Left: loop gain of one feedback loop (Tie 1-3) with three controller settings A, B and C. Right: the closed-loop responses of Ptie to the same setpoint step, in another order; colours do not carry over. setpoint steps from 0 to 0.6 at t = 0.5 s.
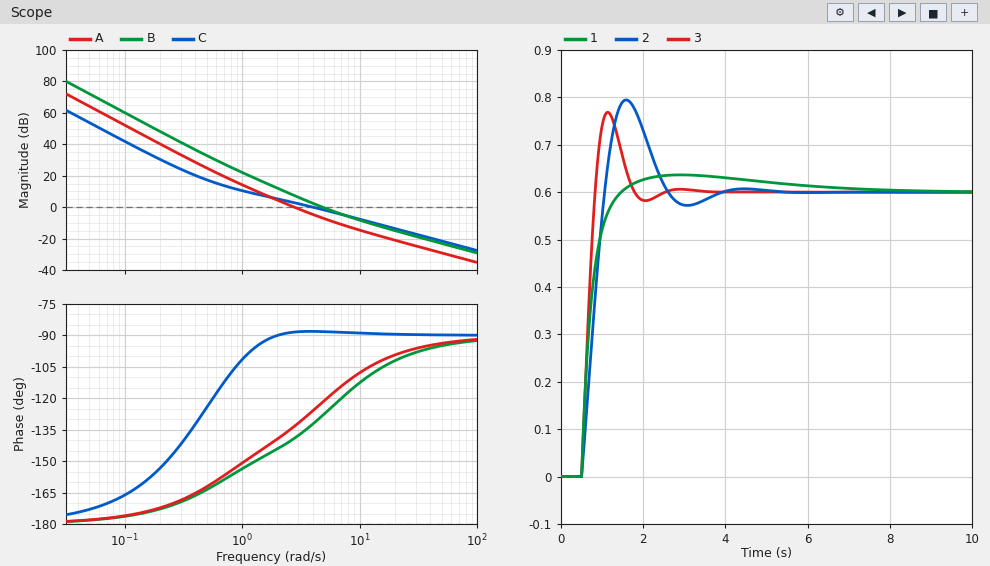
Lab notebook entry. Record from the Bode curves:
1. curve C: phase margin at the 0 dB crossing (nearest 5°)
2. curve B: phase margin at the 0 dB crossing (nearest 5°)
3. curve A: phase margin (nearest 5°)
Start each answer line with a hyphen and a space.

- 90°
- 50°
- 45°
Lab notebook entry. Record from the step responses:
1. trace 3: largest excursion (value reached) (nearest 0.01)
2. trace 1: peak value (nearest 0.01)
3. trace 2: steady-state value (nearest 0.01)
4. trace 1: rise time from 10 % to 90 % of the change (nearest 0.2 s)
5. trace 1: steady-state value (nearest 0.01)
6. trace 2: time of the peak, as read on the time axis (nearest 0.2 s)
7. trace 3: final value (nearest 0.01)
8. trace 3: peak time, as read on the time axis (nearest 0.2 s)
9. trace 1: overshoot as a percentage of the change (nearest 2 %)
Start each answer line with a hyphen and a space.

- 0.77
- 0.64
- 0.60
- 0.6 s
- 0.60
- 1.6 s
- 0.60
- 1.2 s
- 6 %
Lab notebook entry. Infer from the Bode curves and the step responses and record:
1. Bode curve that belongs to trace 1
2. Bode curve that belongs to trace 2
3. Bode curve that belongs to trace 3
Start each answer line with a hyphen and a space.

- C
- A
- B
